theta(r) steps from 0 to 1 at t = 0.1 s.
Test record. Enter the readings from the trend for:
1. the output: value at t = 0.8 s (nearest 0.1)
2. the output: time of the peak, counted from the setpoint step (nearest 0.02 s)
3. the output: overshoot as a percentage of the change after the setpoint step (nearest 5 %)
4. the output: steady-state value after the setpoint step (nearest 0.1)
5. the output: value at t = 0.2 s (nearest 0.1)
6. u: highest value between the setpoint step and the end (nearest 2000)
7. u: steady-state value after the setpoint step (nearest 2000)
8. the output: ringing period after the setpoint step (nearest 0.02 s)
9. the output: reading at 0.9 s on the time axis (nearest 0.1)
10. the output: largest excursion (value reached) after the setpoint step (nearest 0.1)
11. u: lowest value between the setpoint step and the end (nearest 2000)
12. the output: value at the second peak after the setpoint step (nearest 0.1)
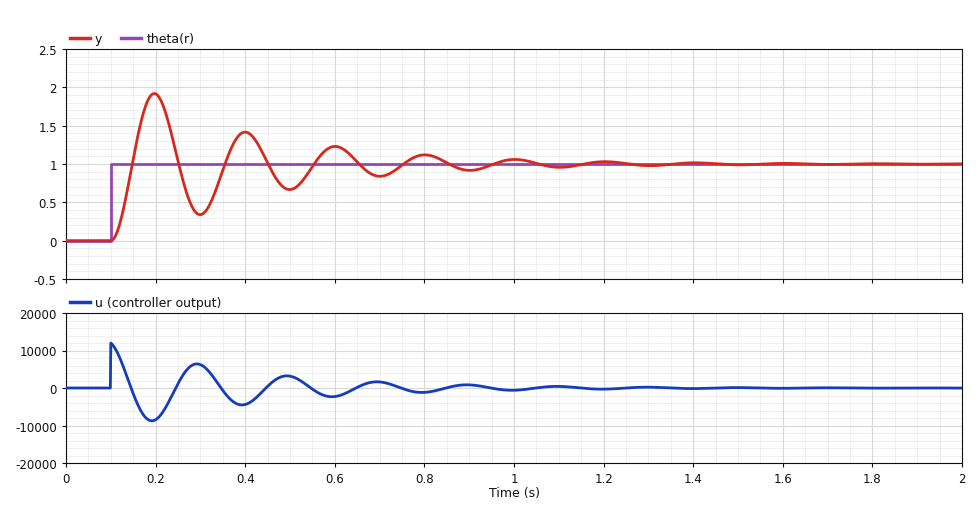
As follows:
1.1
0.10 s
90 %
1.0
1.9
12000
0
0.20 s
0.9
1.9
-8000
1.4
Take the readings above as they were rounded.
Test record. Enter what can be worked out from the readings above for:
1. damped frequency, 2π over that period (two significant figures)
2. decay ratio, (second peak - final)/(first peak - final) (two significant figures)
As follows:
31 rad/s
0.44
